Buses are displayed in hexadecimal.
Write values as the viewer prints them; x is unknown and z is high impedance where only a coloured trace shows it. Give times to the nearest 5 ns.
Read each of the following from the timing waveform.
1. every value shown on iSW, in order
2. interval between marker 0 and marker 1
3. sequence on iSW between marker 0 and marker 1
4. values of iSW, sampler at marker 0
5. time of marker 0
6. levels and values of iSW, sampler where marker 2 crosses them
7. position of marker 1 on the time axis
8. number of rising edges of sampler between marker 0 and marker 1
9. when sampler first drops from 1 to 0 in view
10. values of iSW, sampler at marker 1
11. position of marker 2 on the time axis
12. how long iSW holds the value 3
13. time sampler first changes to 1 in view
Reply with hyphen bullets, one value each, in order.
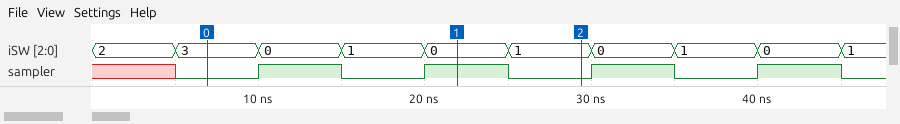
- 2, 3, 0, 1, 0, 1, 0, 1, 0, 1
- 15 ns
- 3, 0, 1, 0
- iSW=3, sampler=0
- 5 ns
- iSW=1, sampler=0
- 20 ns
- 2
- 15 ns
- iSW=0, sampler=1
- 30 ns
- 5 ns
- 10 ns
